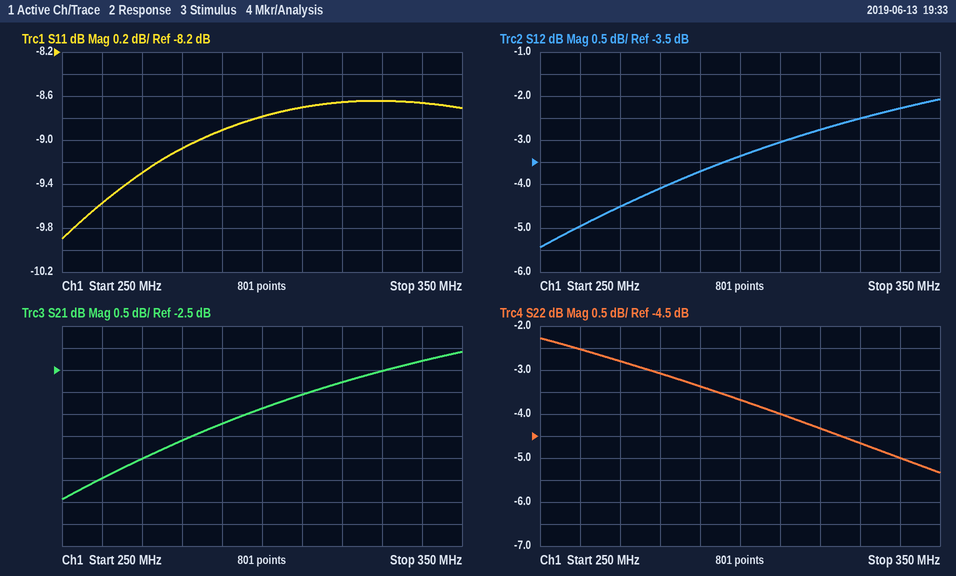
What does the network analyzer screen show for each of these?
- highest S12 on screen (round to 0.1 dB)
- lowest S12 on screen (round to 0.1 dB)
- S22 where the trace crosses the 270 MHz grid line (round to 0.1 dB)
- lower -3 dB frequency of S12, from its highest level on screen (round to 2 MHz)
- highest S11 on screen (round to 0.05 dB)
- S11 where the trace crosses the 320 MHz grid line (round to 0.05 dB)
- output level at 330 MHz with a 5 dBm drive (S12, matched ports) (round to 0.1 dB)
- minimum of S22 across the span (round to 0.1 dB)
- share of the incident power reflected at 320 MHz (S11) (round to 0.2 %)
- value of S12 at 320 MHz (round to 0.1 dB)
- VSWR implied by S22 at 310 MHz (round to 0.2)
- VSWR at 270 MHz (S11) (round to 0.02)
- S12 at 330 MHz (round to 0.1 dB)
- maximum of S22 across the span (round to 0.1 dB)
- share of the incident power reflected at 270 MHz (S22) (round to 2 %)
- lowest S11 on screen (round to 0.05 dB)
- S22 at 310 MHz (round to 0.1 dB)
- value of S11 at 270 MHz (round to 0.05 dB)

-2.1 dB
-5.4 dB
-2.8 dB
258 MHz
-8.65 dB
-8.65 dB
2.5 dBm
-5.3 dB
13.6 %
-2.8 dB
4.4
2.04
-2.5 dB
-2.3 dB
52 %
-9.90 dB
-4.0 dB
-9.30 dB
